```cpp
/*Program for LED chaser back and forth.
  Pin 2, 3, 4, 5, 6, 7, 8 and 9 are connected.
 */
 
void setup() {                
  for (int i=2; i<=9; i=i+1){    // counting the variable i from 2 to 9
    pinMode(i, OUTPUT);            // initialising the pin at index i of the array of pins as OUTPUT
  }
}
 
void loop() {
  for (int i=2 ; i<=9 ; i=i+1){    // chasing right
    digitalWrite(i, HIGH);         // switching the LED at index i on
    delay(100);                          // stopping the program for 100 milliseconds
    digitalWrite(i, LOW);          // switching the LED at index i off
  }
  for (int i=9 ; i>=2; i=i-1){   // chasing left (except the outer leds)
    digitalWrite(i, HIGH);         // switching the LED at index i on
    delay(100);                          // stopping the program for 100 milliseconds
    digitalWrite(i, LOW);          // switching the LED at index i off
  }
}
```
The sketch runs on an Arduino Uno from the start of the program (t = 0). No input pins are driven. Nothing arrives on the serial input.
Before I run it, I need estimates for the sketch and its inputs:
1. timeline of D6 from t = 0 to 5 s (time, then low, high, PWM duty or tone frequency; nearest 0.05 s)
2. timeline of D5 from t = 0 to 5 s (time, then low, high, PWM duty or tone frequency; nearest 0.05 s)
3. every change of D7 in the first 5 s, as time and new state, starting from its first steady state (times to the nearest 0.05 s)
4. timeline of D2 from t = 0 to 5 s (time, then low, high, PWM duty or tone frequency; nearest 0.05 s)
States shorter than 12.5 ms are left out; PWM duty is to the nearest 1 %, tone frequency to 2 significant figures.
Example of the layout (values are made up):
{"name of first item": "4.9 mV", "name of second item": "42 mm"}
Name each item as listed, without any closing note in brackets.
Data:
{"timeline of D6 from t = 0 to 5 s": "0 s low; 0.4 s high; 0.5 s low; 1.1 s high; 1.2 s low; 2 s high; 2.1 s low; 2.7 s high; 2.8 s low; 3.6 s high; 3.7 s low; 4.3 s high; 4.4 s low", "timeline of D5 from t = 0 to 5 s": "0 s low; 0.3 s high; 0.4 s low; 1.2 s high; 1.3 s low; 1.9 s high; 2 s low; 2.8 s high; 2.9 s low; 3.5 s high; 3.6 s low; 4.4 s high; 4.5 s low", "every change of D7 in the first 5 s, as time and new state, starting from its first steady state": "0 s low; 0.5 s high; 0.6 s low; 1 s high; 1.1 s low; 2.1 s high; 2.2 s low; 2.6 s high; 2.7 s low; 3.7 s high; 3.8 s low; 4.2 s high; 4.3 s low", "timeline of D2 from t = 0 to 5 s": "0 s high; 0.1 s low; 1.5 s high; 1.7 s low; 3.1 s high; 3.3 s low; 4.7 s high; 4.9 s low"}
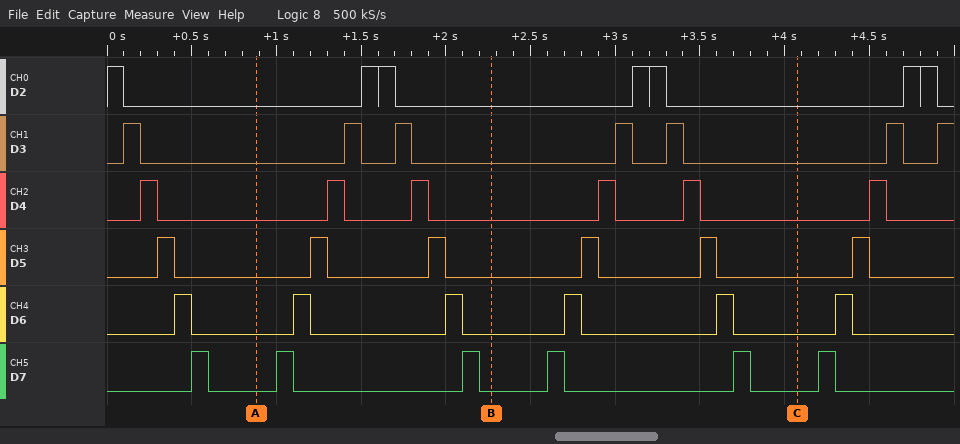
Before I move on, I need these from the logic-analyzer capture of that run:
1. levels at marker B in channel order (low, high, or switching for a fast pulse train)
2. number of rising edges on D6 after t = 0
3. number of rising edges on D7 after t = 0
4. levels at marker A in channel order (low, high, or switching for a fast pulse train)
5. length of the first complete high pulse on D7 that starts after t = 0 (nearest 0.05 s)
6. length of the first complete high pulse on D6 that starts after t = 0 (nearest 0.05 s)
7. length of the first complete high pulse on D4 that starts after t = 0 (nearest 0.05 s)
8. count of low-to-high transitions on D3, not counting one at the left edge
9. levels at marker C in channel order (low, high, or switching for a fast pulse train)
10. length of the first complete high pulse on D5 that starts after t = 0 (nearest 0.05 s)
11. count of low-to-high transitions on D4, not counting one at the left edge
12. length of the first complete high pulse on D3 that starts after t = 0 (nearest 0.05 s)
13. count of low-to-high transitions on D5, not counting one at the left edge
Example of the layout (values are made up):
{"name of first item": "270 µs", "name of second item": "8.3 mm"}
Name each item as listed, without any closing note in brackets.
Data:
{"levels at marker B in channel order": "D2 low, D3 low, D4 low, D5 low, D6 low, D7 low", "number of rising edges on D6 after t = 0": "6", "number of rising edges on D7 after t = 0": "6", "levels at marker A in channel order": "D2 low, D3 low, D4 low, D5 low, D6 low, D7 low", "length of the first complete high pulse on D7 that starts after t = 0": "0.10 s", "length of the first complete high pulse on D6 that starts after t = 0": "0.10 s", "length of the first complete high pulse on D4 that starts after t = 0": "0.10 s", "count of low-to-high transitions on D3, not counting one at the left edge": "7", "levels at marker C in channel order": "D2 low, D3 low, D4 low, D5 low, D6 low, D7 low", "length of the first complete high pulse on D5 that starts after t = 0": "0.10 s", "count of low-to-high transitions on D4, not counting one at the left edge": "6", "length of the first complete high pulse on D3 that starts after t = 0": "0.10 s", "count of low-to-high transitions on D5, not counting one at the left edge": "6"}
